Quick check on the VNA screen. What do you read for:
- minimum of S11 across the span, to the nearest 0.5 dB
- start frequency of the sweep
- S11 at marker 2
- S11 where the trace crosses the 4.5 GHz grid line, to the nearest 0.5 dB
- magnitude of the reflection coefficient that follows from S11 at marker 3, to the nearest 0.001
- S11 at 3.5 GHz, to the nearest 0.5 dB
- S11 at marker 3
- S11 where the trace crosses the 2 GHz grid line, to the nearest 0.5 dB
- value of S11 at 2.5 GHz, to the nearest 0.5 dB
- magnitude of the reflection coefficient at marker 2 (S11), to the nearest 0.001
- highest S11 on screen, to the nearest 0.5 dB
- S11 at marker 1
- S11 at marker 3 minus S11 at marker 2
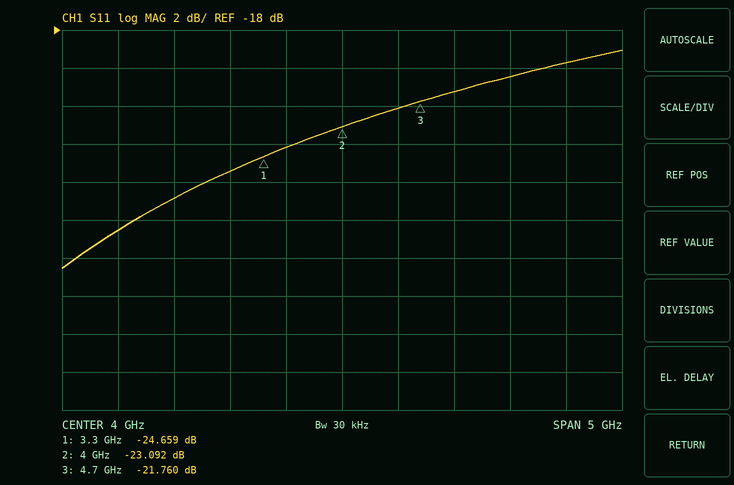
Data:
-30.5 dB
1.5 GHz
-23.092 dB
-22.0 dB
0.082
-24.0 dB
-21.760 dB
-28.5 dB
-27.0 dB
0.070
-19.0 dB
-24.659 dB
1.332 dB
